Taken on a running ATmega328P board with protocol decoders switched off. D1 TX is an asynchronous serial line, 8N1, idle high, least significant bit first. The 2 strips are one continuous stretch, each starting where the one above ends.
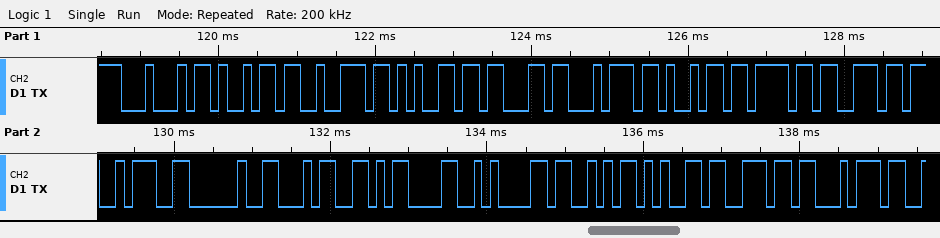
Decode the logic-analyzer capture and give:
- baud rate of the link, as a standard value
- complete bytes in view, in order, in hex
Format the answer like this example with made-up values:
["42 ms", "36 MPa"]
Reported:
["9600 baud", "0x44 0x69 0x72 0x65 0x63 0x74 0x69 0x6F 0x6E 0x3A 0x20 0x34 0x0D 0x0A 0x53 0x65 0x6E 0x74"]
